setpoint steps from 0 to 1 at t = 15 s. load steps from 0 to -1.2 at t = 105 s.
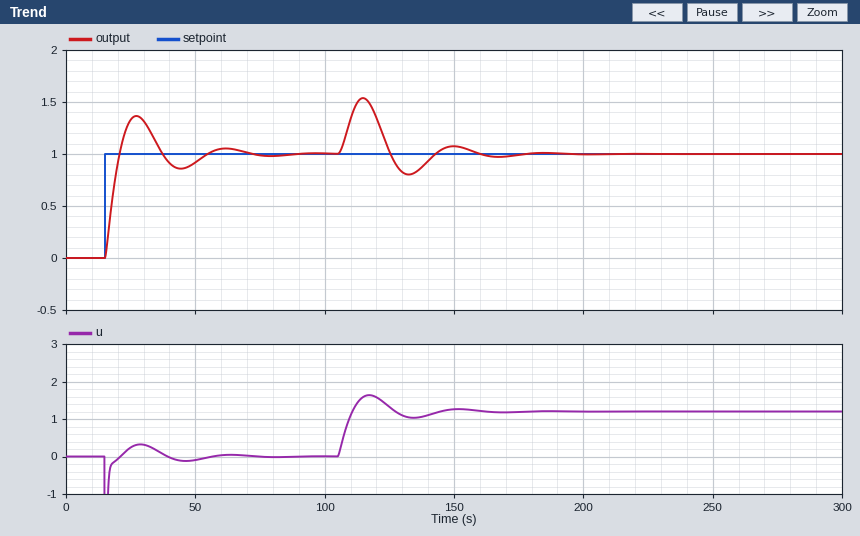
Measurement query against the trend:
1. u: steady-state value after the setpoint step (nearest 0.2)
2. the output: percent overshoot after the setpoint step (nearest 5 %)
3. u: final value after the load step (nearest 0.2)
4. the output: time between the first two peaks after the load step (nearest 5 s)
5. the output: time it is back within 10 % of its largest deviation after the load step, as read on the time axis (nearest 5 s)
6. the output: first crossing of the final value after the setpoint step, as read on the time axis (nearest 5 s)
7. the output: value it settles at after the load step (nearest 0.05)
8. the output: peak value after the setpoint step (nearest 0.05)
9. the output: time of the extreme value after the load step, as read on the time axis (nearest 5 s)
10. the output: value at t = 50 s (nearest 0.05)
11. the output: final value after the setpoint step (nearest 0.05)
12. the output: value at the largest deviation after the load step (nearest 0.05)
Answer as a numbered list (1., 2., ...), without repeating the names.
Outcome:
1. 0.0
2. 35 %
3. 1.2
4. 35 s
5. 155 s
6. 20 s
7. 1.00
8. 1.35
9. 115 s
10. 0.90
11. 1.00
12. 1.55
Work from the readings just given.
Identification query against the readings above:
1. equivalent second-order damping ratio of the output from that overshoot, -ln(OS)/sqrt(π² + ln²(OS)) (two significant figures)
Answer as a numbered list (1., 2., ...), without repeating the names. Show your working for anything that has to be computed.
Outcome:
1. ln(0.35) = -1.050; 1.050 / sqrt(9.870 + 1.102) = 0.32
